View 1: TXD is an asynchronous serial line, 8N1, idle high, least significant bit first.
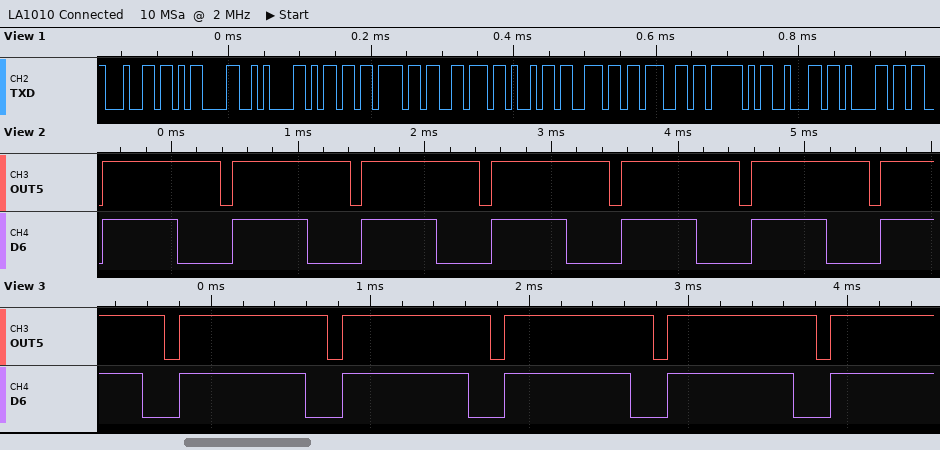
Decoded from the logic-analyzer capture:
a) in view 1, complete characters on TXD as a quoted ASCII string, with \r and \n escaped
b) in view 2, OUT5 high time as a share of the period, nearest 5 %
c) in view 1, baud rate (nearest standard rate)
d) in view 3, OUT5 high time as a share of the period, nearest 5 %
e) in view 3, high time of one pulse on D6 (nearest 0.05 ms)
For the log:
"d\r\nmoving_ba"
90 %
115200 baud
90 %
0.80 ms
